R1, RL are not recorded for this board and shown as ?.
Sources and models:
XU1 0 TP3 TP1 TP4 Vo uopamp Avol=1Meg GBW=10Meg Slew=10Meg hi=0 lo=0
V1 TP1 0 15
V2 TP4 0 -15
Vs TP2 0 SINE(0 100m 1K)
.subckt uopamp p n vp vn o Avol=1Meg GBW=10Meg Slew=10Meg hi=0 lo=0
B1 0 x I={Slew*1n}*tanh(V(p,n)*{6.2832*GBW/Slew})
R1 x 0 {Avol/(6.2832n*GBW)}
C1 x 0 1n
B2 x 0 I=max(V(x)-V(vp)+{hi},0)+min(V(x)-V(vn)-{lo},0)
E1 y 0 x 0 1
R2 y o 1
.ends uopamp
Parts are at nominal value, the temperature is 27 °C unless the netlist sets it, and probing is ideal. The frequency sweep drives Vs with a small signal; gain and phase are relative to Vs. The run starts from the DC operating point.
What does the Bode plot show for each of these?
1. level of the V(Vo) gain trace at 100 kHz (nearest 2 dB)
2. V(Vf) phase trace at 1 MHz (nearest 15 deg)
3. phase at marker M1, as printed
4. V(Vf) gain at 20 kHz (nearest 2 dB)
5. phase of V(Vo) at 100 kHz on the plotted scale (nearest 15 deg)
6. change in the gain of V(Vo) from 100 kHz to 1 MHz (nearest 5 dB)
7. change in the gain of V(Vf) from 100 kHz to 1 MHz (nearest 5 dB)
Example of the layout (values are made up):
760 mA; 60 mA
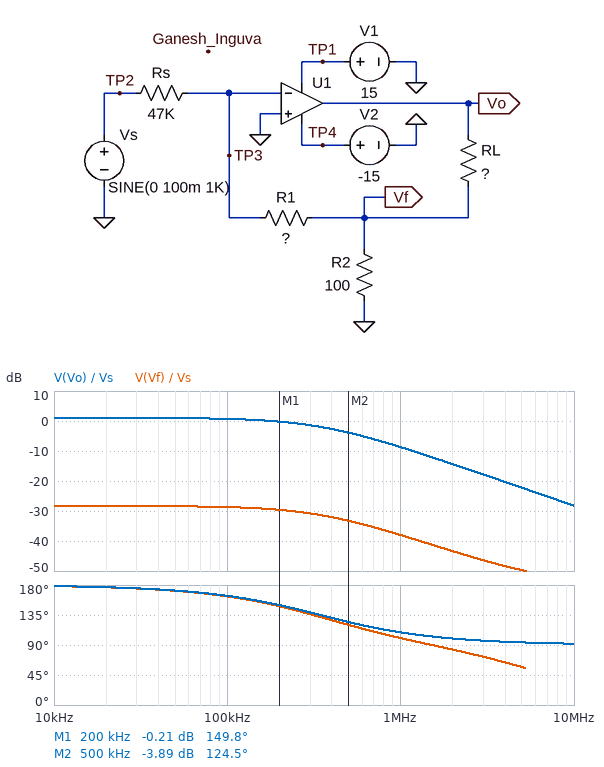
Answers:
0 dB; 105 deg; 149.8 deg; -28 dB; 165 deg; -10 dB; -10 dB
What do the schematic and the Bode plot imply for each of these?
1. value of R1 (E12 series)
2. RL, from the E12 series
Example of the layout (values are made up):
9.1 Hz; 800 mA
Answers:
1.8 kΩ; 2.7 kΩ
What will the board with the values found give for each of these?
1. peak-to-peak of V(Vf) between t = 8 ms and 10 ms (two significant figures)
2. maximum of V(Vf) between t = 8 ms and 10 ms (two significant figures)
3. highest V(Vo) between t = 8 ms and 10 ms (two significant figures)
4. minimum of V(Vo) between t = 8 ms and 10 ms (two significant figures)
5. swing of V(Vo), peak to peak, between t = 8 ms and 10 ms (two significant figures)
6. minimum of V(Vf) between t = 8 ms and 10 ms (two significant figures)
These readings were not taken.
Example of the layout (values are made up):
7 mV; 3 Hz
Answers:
7.7 mV; 3.8 mV; 110 mV; -110 mV; 230 mV; -3.8 mV
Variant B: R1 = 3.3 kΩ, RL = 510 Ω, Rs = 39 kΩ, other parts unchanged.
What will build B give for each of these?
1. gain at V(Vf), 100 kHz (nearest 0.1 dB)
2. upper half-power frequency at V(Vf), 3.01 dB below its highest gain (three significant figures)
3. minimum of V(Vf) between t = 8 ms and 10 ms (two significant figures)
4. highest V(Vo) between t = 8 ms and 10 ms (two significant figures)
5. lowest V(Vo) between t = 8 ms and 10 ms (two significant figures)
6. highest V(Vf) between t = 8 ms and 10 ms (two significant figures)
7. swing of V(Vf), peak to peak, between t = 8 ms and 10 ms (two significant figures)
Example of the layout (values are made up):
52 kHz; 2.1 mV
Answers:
-21.5 dB; 1.51 MHz; -8.5 mV; 53 mV; -53 mV; 8.5 mV; 17 mV
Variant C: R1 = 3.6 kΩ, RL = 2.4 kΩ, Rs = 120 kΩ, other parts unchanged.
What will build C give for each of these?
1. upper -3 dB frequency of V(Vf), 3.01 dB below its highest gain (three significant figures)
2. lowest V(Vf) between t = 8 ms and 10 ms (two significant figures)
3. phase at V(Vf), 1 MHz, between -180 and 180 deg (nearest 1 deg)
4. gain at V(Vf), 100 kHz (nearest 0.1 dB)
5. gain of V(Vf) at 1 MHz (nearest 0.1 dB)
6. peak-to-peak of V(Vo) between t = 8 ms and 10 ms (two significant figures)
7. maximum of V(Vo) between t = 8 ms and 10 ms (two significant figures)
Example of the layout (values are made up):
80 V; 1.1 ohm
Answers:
388 kHz; -3.0 mV; 107 deg; -30.7 dB; -39.3 dB; 150 mV; 77 mV
